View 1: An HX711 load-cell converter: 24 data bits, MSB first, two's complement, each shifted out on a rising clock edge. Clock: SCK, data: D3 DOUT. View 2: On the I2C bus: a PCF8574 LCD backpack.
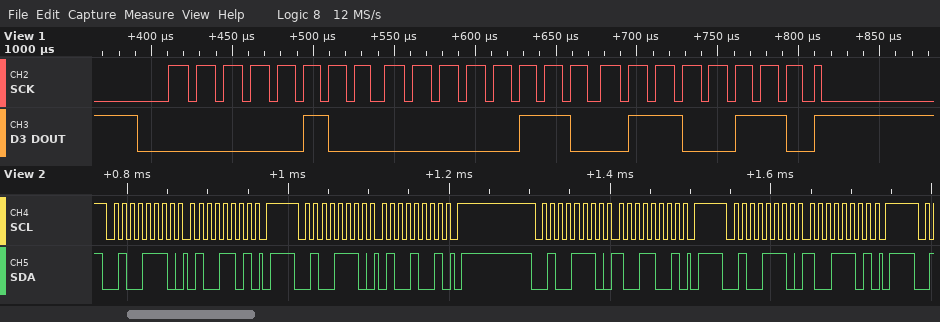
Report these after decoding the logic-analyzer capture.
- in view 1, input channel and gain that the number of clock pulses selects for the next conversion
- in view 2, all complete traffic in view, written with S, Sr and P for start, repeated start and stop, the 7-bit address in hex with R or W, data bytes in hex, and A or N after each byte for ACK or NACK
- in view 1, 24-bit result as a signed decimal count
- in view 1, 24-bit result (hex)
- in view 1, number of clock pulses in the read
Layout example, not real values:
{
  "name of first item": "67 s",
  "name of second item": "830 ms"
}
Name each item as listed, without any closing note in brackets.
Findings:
{
  "in view 1, input channel and gain that the number of clock pulses selects for the next conversion": "channel A, gain 128",
  "in view 2, all complete traffic in view, written with S, Sr and P for start, repeated start and stop, the 7-bit address in hex with R or W, data bytes in hex, and A or N after each byte for ACK or NACK": "S 27W A 4D A P S 27W A 49 A P S 27W A 99 A P S 27W A 9D A P",
  "in view 1, 24-bit result as a signed decimal count": "263782",
  "in view 1, 24-bit result": "0x040666",
  "in view 1, number of clock pulses in the read": "25"
}
